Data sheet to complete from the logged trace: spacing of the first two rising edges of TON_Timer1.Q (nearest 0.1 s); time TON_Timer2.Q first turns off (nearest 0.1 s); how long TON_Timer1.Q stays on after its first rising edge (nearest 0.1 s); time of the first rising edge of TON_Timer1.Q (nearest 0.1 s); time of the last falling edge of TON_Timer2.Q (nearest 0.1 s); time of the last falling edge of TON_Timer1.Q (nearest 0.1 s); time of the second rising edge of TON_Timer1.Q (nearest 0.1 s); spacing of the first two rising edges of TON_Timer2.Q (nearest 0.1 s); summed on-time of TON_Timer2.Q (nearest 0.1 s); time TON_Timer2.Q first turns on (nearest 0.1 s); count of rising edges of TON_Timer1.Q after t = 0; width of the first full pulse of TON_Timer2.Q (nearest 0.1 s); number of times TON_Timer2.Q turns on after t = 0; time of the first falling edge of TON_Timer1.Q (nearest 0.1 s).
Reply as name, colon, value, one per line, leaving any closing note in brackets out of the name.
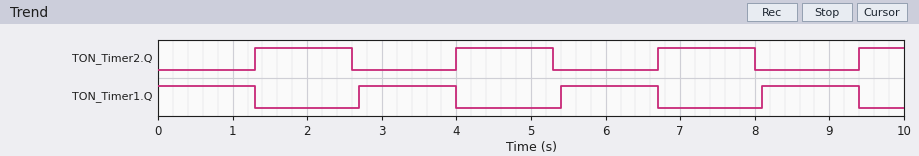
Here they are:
spacing of the first two rising edges of TON_Timer1.Q: 2.7 s
time TON_Timer2.Q first turns off: 2.6 s
how long TON_Timer1.Q stays on after its first rising edge: 1.3 s
time of the first rising edge of TON_Timer1.Q: 2.7 s
time of the last falling edge of TON_Timer2.Q: 8.0 s
time of the last falling edge of TON_Timer1.Q: 9.4 s
time of the second rising edge of TON_Timer1.Q: 5.4 s
spacing of the first two rising edges of TON_Timer2.Q: 2.7 s
summed on-time of TON_Timer2.Q: 4.5 s
time TON_Timer2.Q first turns on: 1.3 s
count of rising edges of TON_Timer1.Q after t = 0: 3
width of the first full pulse of TON_Timer2.Q: 1.3 s
number of times TON_Timer2.Q turns on after t = 0: 4
time of the first falling edge of TON_Timer1.Q: 1.3 s
